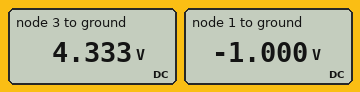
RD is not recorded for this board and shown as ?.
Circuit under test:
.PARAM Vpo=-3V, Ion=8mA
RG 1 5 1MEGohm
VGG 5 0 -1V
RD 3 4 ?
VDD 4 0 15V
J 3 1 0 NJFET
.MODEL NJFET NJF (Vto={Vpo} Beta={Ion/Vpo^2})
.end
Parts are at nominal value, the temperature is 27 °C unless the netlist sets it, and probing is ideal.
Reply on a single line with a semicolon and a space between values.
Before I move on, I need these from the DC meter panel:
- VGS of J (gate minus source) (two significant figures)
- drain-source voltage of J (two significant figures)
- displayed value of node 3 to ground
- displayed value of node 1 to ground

-1.0 V; 4.3 V; 4.333 V; -1.000 V
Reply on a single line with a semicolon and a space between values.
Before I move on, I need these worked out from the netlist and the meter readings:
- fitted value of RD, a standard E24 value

3 kΩ
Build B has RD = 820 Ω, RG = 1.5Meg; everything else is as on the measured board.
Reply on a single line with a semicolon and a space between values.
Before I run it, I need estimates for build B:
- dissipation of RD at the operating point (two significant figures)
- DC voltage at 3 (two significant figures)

10 mW; 12 V
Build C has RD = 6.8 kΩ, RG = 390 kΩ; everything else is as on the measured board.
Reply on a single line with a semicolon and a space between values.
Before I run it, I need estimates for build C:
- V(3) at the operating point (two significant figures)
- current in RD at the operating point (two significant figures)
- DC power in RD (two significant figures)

720 mV; 2.1 mA; 30 mW
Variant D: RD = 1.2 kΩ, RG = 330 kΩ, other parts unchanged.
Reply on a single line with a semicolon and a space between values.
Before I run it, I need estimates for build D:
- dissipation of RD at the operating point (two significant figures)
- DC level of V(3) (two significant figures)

15 mW; 11 V
